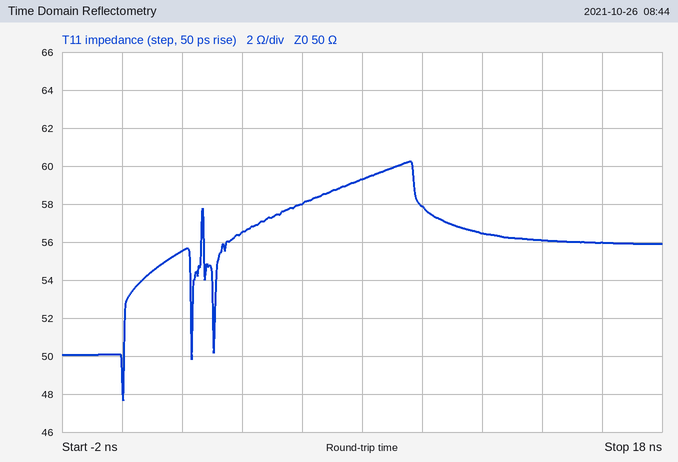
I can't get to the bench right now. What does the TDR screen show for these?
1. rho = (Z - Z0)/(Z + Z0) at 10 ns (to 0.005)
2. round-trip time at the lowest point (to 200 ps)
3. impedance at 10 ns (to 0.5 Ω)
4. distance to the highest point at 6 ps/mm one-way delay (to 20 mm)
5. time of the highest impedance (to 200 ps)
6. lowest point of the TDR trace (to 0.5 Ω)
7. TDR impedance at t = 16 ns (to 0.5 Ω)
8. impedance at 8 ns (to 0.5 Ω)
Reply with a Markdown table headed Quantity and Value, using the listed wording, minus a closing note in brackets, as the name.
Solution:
| Quantity | Value |
|---|---|
| rho = (Z - Z0)/(Z + Z0) at 10 ns | +0.075 |
| round-trip time at the lowest point | 0.0 ns |
| impedance at 10 ns | 58.0 Ω |
| distance to the highest point at 6 ps/mm one-way delay | 800 mm |
| time of the highest impedance | 9.6 ns |
| lowest point of the TDR trace | 47.5 Ω |
| TDR impedance at t = 16 ns | 56.0 Ω |
| impedance at 8 ns | 59.5 Ω |
